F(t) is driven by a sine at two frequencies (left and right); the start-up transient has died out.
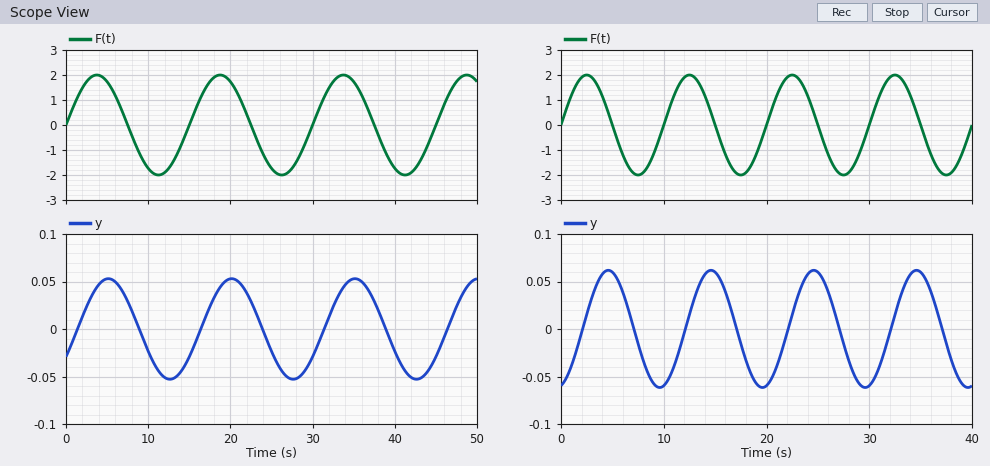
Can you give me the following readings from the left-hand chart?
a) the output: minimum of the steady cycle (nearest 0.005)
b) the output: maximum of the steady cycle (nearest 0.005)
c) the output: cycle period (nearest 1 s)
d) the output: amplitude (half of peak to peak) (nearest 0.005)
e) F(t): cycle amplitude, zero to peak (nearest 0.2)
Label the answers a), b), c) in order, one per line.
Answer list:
a) -0.055
b) 0.055
c) 15 s
d) 0.055
e) 2.0
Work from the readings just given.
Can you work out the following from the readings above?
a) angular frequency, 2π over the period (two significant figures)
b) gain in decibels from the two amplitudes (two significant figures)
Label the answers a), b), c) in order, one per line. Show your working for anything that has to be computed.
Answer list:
a) 2π / 15 = 0.42 rad/s
b) 20 log10(0.055 / 2) = -31 dB
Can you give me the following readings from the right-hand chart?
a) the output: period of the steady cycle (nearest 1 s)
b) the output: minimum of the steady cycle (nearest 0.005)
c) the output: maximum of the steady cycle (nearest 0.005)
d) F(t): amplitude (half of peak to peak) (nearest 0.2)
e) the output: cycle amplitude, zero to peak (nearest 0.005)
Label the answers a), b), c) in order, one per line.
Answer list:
a) 10 s
b) -0.060
c) 0.060
d) 2.0
e) 0.060
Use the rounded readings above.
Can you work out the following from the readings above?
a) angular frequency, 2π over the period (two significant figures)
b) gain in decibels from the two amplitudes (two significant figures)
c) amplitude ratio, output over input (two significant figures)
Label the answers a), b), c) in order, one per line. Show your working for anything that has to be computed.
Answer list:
a) 2π / 10 = 0.63 rad/s
b) 20 log10(0.06 / 2) = -30 dB
c) 0.06 / 2 = 0.030
